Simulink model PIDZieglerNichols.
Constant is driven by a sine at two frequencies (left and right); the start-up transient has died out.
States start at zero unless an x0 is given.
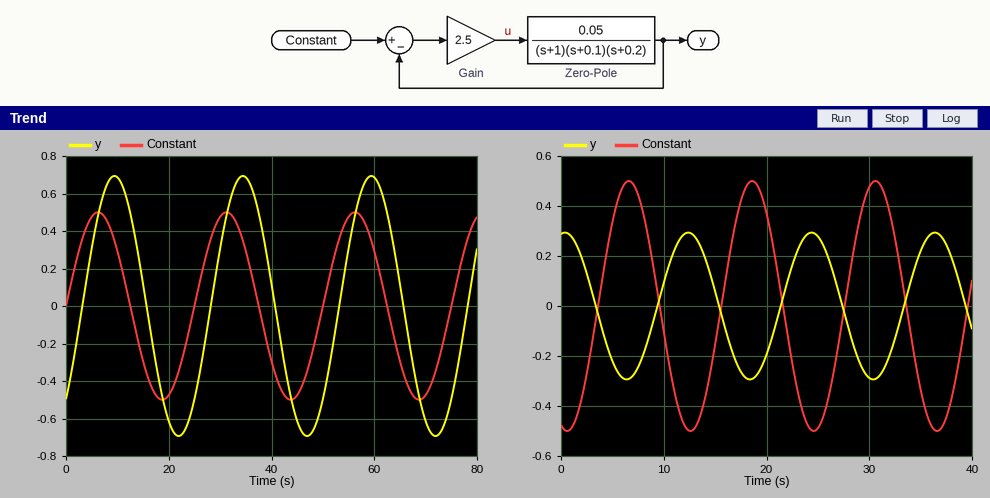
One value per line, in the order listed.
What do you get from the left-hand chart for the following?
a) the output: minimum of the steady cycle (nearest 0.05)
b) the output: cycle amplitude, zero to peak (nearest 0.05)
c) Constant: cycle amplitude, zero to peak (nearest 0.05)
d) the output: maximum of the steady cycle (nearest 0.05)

-0.70
0.70
0.50
0.70
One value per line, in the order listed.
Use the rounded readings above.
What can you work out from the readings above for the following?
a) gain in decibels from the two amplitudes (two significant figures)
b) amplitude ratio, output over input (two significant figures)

2.9 dB
1.4
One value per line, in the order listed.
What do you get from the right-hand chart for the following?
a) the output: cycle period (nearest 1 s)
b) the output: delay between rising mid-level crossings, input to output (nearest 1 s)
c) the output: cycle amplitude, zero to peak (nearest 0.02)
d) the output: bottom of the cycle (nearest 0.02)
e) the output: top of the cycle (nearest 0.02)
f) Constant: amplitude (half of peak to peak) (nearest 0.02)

12 s
6 s
0.30
-0.30
0.30
0.50
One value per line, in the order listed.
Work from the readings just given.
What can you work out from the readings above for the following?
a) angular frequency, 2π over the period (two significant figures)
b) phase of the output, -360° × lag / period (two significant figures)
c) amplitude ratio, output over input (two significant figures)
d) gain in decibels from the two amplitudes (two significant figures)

0.52 rad/s
-180°
0.60
-4.4 dB
